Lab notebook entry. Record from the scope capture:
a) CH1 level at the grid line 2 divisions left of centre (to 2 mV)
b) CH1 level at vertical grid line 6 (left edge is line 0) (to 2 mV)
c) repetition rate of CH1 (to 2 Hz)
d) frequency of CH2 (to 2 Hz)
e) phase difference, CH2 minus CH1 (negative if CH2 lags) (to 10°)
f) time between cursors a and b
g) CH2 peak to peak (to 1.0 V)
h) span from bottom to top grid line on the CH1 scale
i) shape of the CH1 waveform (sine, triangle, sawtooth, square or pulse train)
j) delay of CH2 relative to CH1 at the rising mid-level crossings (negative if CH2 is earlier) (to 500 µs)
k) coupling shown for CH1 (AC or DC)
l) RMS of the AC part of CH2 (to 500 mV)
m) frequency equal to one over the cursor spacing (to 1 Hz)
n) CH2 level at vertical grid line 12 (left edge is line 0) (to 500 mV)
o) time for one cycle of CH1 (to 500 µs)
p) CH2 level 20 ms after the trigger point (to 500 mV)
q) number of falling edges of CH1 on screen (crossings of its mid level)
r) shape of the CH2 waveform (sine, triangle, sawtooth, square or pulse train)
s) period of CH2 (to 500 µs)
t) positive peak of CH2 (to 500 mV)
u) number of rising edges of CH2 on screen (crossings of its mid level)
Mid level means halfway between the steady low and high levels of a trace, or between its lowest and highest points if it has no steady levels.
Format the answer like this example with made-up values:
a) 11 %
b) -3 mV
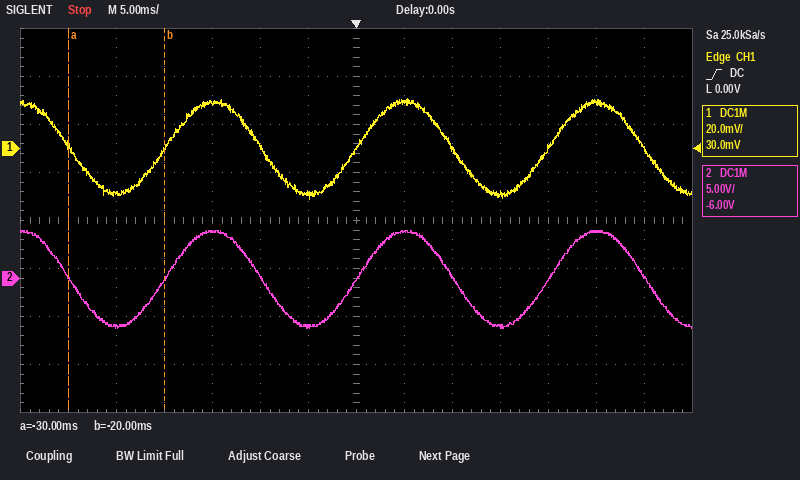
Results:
a) 2 mV
b) -20 mV
c) 50 Hz
d) 50 Hz
e) 0°
f) 10.0 ms
g) 10.0 V
h) 160 mV
i) sine
j) 0.0 ms
k) DC
l) 3.5 V
m) 100 Hz
n) 5.0 V
o) 20.0 ms
p) 0.0 V
q) 4
r) sine
s) 20.0 ms
t) 5.0 V
u) 3
